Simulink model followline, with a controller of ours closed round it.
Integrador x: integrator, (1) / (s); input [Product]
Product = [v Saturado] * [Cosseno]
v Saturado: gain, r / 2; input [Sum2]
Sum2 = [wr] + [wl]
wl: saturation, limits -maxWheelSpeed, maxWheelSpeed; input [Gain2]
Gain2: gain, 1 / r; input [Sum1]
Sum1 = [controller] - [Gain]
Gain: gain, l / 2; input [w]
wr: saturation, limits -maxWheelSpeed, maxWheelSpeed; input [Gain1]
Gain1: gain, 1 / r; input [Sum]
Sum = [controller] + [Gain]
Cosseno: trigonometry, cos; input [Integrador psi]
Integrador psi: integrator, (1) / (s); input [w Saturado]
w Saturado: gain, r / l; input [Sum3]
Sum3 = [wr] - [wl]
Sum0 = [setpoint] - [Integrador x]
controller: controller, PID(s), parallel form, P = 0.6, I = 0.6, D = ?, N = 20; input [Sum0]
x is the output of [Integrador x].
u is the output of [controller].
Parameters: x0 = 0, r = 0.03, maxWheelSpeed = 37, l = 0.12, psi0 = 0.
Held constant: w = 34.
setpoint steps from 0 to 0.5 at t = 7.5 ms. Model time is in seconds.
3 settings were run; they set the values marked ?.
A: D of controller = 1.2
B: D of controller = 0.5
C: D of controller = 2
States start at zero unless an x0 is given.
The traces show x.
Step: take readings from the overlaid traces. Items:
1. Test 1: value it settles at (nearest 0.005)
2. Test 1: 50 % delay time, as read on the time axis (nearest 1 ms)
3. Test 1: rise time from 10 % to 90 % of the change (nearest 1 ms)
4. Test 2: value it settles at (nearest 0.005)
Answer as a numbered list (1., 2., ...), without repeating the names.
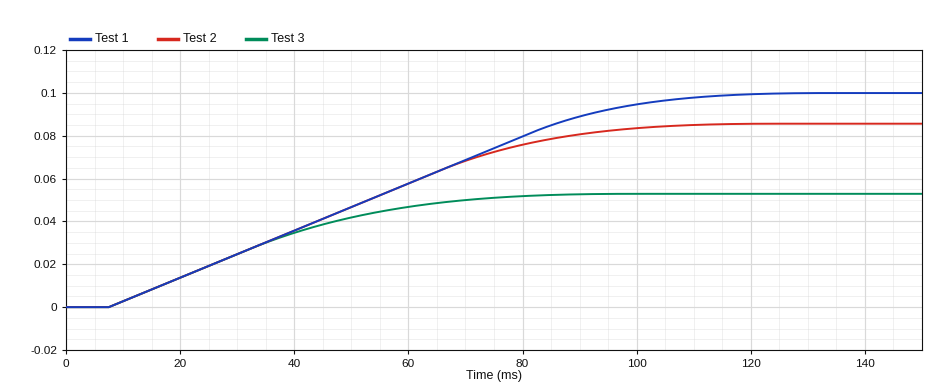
1. 0.100
2. 53 ms
3. 75 ms
4. 0.085
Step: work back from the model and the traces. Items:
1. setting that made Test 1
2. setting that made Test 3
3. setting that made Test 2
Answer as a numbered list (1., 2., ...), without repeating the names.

1. C
2. B
3. A
